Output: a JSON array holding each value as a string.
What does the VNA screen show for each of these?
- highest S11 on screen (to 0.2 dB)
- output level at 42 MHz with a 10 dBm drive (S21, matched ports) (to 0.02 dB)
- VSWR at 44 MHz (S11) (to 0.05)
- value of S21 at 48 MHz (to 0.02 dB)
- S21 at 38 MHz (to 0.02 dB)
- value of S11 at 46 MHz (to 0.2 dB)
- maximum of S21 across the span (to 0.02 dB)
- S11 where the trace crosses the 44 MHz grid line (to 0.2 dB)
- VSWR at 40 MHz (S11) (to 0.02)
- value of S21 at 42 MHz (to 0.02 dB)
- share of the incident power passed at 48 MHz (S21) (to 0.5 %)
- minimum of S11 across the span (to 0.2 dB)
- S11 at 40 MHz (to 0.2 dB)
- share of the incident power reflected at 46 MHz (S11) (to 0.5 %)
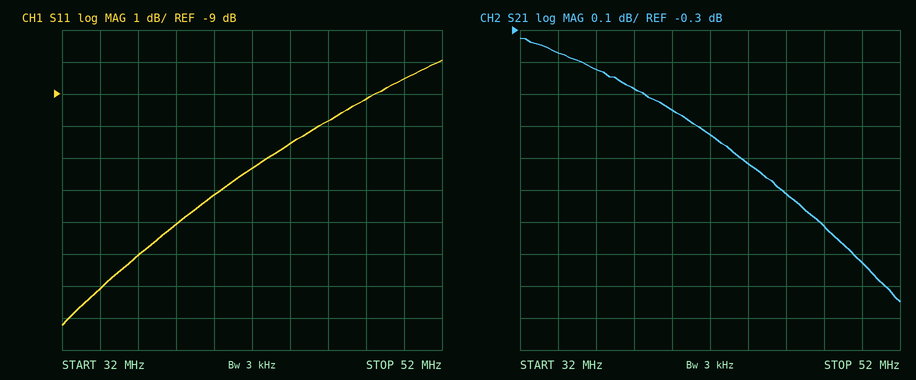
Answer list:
["-8.0 dB", "9.38 dBm", "1.85", "-0.92 dB", "-0.48 dB", "-9.8 dB", "-0.32 dB", "-10.6 dB", "1.66", "-0.62 dB", "81.0 %", "-16.2 dB", "-12.2 dB", "10.5 %"]
